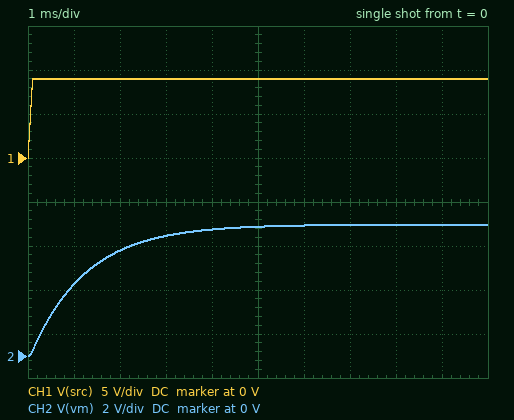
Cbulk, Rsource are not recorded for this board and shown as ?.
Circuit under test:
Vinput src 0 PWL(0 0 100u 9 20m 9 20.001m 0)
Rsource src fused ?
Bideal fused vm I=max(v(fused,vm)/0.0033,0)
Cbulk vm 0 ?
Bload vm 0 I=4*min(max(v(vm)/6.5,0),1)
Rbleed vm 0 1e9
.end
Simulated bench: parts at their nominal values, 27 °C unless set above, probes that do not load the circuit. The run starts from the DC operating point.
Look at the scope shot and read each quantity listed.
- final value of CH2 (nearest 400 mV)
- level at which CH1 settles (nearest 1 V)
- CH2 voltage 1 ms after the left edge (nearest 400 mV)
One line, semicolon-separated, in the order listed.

6.0 V; 9 V; 3.2 V
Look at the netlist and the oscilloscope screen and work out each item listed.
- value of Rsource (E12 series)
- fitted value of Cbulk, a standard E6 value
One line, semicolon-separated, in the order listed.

0.82 Ω; 2.2 mF
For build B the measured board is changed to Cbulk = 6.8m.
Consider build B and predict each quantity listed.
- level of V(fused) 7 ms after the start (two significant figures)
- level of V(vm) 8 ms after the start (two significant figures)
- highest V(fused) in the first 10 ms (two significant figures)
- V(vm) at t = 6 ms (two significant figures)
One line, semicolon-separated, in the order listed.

5.1 V; 5.3 V; 5.6 V; 4.8 V
